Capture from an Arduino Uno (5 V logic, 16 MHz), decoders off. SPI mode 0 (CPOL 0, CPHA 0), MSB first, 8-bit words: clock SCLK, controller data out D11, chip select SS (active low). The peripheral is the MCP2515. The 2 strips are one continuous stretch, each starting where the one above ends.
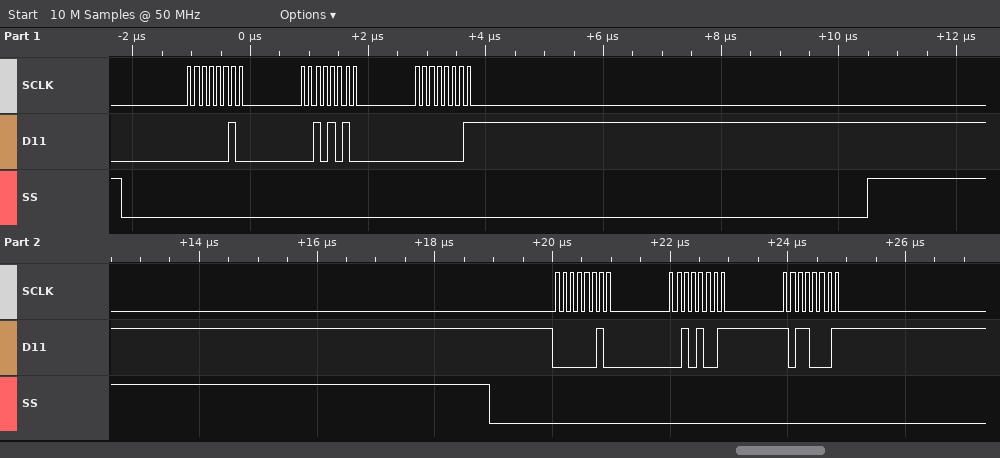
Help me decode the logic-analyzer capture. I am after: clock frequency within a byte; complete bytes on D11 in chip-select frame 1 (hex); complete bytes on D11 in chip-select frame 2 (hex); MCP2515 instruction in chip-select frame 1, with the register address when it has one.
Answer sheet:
8 MHz
0x02 0x2A 0x01
0x02 0x29 0xB1
WRITE 0x2A
